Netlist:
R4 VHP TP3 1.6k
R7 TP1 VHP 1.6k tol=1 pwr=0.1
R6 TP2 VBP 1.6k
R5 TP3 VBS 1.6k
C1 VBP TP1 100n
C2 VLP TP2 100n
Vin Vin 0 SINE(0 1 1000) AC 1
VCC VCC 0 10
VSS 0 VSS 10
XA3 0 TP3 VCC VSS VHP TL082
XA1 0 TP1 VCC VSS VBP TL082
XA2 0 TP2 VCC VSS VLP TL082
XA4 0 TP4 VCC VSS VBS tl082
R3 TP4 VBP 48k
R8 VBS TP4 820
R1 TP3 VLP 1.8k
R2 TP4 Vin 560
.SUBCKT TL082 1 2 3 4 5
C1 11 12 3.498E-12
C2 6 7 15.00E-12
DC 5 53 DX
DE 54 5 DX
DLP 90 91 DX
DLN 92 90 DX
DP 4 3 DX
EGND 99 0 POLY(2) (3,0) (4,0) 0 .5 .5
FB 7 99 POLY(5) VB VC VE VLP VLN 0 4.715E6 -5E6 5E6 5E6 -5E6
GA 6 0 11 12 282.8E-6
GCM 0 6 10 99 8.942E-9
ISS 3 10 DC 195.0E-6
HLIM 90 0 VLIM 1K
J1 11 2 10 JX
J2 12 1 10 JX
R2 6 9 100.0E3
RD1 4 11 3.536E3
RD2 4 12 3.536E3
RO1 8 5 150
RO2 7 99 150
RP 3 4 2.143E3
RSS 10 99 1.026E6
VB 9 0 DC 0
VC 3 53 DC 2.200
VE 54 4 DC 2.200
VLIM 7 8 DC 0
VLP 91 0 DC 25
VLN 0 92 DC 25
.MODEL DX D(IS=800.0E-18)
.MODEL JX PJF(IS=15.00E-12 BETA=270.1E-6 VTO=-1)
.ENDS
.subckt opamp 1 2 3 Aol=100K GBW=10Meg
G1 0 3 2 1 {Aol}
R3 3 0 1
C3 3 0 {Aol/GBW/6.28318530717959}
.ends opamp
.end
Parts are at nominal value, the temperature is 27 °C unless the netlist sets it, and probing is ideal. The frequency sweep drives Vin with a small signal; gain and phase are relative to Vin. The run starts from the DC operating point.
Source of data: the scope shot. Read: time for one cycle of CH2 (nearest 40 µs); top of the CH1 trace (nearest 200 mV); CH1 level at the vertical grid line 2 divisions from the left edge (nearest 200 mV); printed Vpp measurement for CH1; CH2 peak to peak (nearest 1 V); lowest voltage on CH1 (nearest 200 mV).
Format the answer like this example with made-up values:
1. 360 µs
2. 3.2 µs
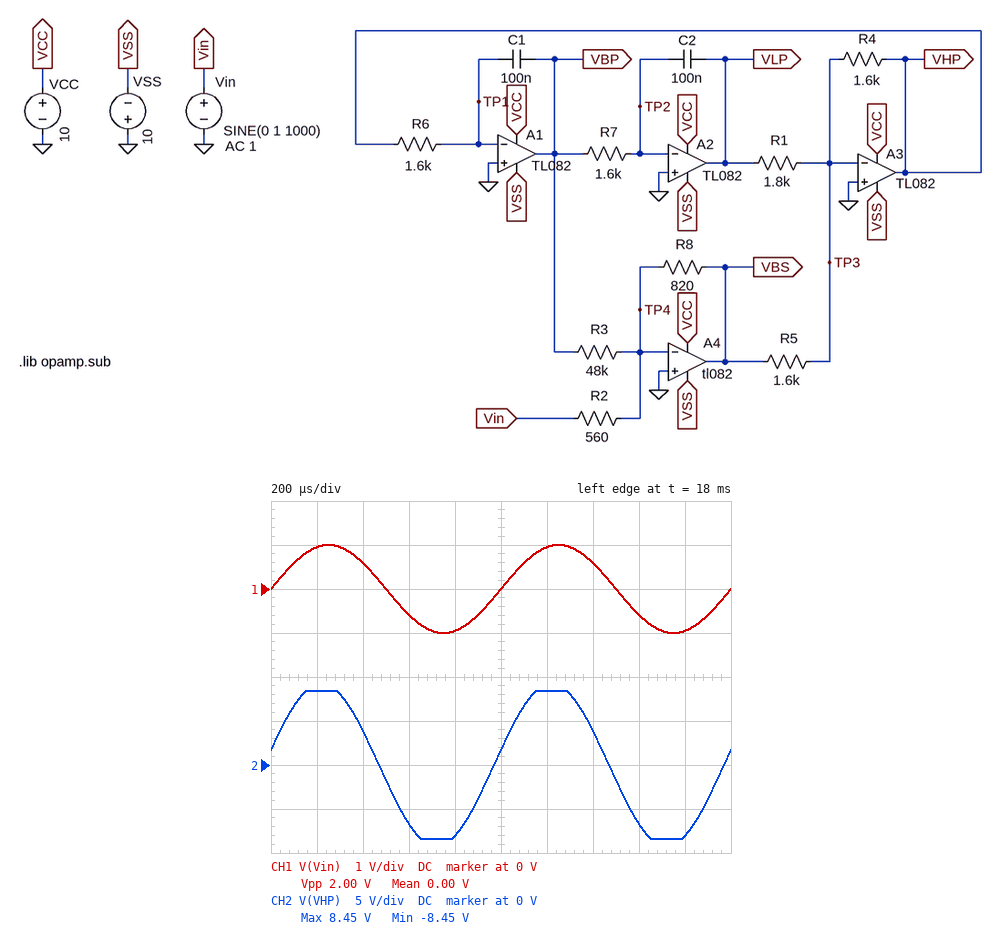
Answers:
1. 1.00 ms
2. 1.0 V
3. 600 mV
4. 2.00 V
5. 17 V
6. -1.0 V
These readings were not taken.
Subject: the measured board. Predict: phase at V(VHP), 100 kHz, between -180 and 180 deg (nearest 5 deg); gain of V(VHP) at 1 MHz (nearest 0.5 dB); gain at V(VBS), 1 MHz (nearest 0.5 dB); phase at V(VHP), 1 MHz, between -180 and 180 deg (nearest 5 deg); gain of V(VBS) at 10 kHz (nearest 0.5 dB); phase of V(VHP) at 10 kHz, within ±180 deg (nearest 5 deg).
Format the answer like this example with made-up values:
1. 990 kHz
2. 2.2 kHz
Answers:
1. -10 deg
2. -0.5 dB
3. 1.5 dB
4. -95 deg
5. 3.5 dB
6. 0 deg
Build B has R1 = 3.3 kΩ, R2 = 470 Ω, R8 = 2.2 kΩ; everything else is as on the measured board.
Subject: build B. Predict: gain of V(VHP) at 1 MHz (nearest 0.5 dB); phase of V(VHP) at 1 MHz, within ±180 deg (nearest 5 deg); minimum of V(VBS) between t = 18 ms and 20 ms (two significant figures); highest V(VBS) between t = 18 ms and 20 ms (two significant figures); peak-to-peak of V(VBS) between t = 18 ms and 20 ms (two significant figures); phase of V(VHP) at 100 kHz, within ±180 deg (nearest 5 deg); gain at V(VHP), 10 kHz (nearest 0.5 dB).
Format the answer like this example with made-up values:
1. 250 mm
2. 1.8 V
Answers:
1. 5.5 dB
2. -115 deg
3. -4.7 V
4. 4.7 V
5. 9.3 V
6. -15 deg
7. 13.5 dB
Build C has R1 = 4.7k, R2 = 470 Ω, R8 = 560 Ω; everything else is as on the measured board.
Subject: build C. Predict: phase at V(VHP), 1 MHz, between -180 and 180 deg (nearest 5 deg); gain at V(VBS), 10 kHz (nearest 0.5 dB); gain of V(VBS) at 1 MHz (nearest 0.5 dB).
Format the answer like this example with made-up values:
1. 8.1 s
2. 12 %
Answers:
1. -90 deg
2. 1.5 dB
3. 0 dB
